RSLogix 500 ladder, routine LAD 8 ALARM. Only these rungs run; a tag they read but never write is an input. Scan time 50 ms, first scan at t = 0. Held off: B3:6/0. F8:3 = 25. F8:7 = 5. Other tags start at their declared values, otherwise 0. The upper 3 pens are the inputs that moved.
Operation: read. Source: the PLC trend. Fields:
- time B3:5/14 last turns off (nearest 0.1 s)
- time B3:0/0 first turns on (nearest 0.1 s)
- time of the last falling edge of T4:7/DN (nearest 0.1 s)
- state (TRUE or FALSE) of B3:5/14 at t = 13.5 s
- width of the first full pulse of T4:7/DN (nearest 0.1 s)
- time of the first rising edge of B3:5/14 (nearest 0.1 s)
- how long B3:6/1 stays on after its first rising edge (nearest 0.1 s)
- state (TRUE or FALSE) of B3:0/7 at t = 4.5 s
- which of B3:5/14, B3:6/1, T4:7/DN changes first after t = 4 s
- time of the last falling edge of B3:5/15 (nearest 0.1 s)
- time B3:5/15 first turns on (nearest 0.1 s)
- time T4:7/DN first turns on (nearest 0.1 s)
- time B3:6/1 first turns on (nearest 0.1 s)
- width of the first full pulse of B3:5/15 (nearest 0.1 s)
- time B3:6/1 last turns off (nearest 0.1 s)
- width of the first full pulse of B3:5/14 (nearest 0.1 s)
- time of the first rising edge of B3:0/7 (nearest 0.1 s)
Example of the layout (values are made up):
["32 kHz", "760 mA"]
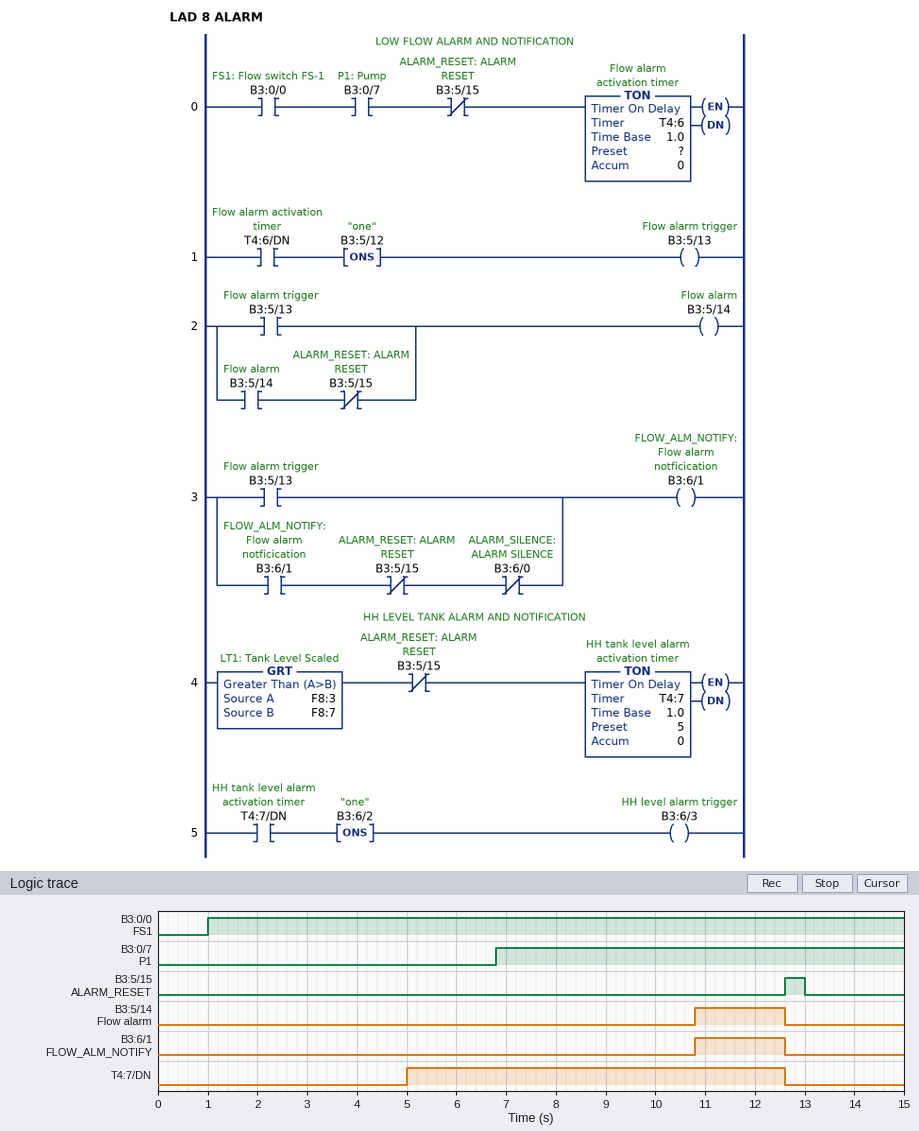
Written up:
["12.6 s", "1.0 s", "12.6 s", "FALSE", "7.6 s", "10.8 s", "1.8 s", "FALSE", "T4:7/DN", "13.0 s", "12.6 s", "5.0 s", "10.8 s", "0.4 s", "12.6 s", "1.8 s", "6.8 s"]
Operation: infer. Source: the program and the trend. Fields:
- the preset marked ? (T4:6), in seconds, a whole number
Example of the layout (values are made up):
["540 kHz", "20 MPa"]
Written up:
["4 s"]
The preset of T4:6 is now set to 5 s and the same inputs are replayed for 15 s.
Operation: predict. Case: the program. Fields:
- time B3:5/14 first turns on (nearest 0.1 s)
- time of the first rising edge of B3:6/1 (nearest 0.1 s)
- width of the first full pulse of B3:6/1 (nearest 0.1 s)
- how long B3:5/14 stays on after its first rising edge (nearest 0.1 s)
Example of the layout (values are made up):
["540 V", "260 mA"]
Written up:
["11.8 s", "11.8 s", "0.8 s", "0.8 s"]
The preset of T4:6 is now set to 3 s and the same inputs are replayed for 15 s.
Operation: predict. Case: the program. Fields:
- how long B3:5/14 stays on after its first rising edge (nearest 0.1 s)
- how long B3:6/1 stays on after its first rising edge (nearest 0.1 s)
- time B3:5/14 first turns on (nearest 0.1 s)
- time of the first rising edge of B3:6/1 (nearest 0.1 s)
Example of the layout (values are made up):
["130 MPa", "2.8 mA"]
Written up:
["2.8 s", "2.8 s", "9.8 s", "9.8 s"]
